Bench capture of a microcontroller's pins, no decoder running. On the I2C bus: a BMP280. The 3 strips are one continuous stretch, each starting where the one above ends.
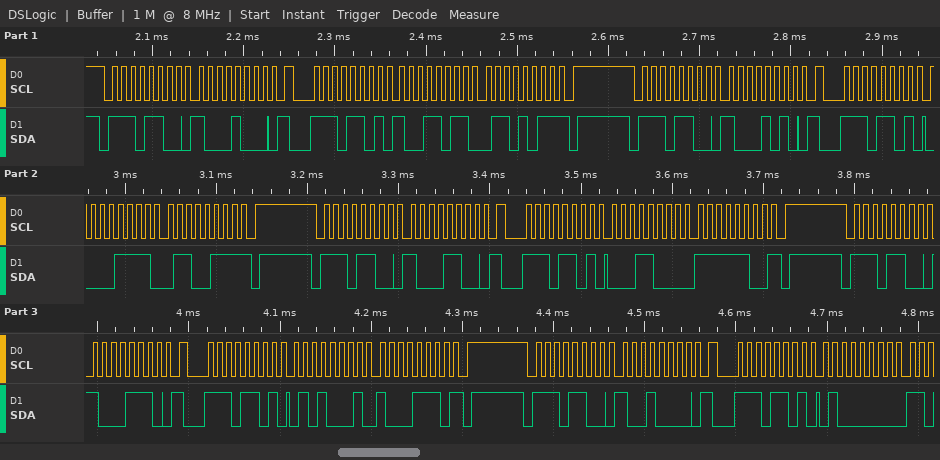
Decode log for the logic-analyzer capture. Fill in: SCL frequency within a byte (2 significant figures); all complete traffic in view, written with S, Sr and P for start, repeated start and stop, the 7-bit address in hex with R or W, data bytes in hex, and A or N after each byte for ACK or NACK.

100 kHz
S 76W A 88 A Sr 76R A 9B A 6B N P S 76W A 8A A Sr 76R A 0F A 67 N P S 76W A 8C A Sr 76R A 18 A FC N P S 76W A 8E A Sr 76R A 51 A 8E N P S 76W A 90 A Sr 76R A 40 A
